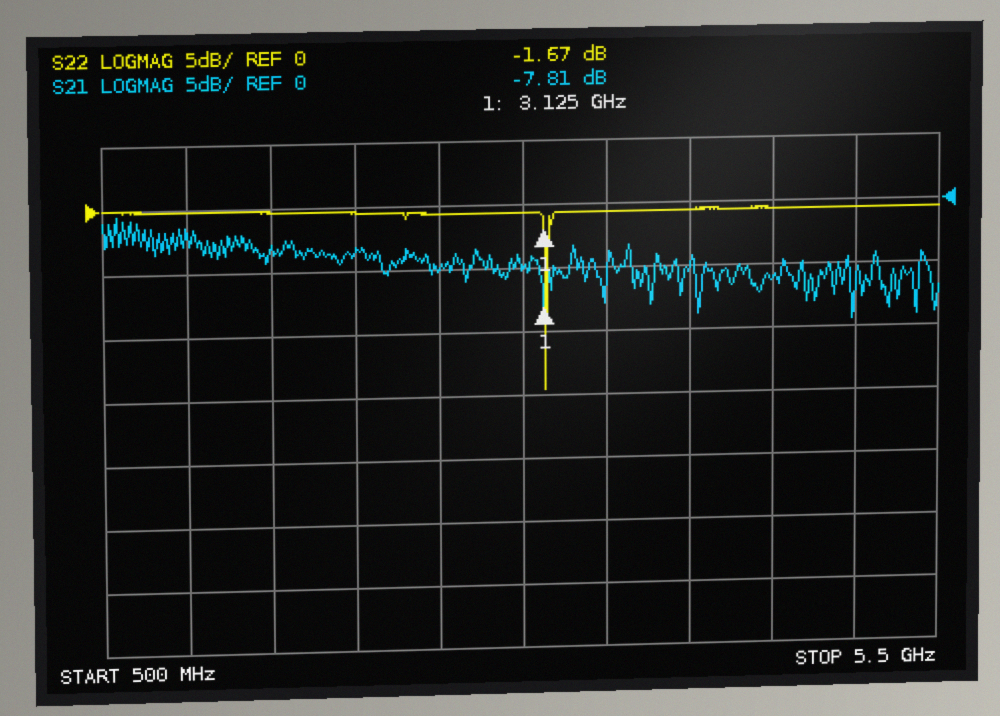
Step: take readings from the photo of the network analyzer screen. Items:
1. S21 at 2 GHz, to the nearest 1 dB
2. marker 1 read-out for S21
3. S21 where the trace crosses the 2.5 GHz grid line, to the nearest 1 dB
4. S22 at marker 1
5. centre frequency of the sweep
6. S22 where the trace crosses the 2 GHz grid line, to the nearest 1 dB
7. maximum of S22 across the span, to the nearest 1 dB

-3 dB
-7.81 dB
-5 dB
-1.67 dB
3 GHz
0 dB
0 dB
